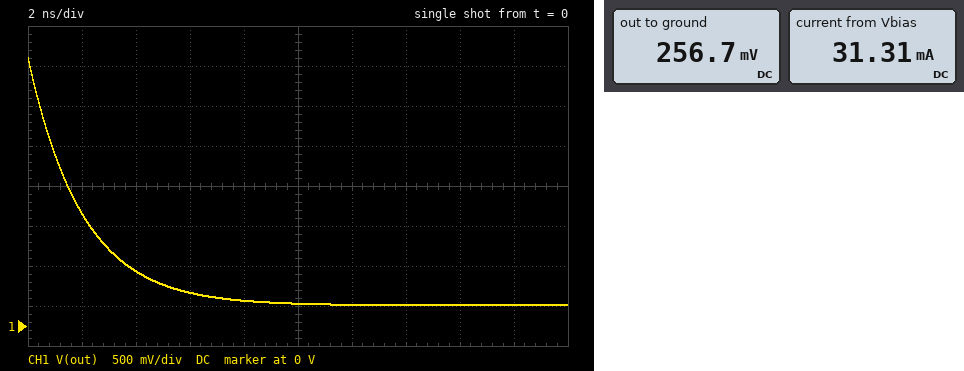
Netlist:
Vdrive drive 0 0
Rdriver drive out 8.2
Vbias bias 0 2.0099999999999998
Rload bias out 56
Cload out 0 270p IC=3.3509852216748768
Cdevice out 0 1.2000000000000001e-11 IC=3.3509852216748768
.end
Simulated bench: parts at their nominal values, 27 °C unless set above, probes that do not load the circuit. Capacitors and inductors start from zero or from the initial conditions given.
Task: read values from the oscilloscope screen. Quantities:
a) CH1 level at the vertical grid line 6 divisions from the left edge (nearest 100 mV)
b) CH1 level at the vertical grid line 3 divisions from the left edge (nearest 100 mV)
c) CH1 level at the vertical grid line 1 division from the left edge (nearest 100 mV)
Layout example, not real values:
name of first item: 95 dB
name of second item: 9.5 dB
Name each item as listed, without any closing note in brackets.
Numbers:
CH1 level at the vertical grid line 6 divisions from the left edge: 300 mV
CH1 level at the vertical grid line 3 divisions from the left edge: 400 mV
CH1 level at the vertical grid line 1 division from the left edge: 1.4 V
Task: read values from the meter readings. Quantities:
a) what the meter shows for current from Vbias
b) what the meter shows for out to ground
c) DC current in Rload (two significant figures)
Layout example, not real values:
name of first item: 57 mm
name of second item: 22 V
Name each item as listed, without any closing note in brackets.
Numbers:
what the meter shows for current from Vbias: 31.31 mA
what the meter shows for out to ground: 256.7 mV
DC current in Rload: 31 mA
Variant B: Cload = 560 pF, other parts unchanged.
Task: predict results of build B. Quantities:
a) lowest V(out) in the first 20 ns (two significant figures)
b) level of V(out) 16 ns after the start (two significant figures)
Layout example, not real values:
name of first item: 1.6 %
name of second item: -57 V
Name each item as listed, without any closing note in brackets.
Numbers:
lowest V(out) in the first 20 ns: 280 mV
level of V(out) 16 ns after the start: 320 mV
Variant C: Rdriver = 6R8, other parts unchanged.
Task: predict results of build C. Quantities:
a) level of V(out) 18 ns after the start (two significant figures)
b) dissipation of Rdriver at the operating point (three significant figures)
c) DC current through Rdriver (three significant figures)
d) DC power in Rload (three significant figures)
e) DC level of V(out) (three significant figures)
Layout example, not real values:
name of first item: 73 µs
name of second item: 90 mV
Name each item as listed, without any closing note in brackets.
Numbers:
level of V(out) 18 ns after the start: 220 mV
dissipation of Rdriver at the operating point: 6.97 mW
DC current through Rdriver: 32.0 mA
DC power in Rload: 57.4 mW
DC level of V(out): 218 mV
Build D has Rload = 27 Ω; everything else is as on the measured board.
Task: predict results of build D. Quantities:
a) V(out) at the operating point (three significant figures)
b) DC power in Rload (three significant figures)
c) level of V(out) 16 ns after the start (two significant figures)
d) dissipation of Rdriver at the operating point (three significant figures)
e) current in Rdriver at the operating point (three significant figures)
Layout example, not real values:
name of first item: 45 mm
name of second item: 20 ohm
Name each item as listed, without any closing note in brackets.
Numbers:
V(out) at the operating point: 468 mV
DC power in Rload: 88.0 mW
level of V(out) 16 ns after the start: 470 mV
dissipation of Rdriver at the operating point: 26.7 mW
current in Rdriver at the operating point: 57.1 mA
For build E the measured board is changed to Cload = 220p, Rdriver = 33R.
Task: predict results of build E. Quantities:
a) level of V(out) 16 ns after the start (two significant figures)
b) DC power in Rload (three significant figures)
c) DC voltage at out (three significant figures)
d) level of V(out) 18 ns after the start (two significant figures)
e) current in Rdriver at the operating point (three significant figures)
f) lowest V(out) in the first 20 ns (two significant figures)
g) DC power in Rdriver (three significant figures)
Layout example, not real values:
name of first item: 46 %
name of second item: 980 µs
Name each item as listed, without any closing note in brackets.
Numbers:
level of V(out) 16 ns after the start: 840 mV
DC power in Rload: 28.6 mW
DC voltage at out: 745 mV
level of V(out) 18 ns after the start: 810 mV
current in Rdriver at the operating point: 22.6 mA
lowest V(out) in the first 20 ns: 790 mV
DC power in Rdriver: 16.8 mW
